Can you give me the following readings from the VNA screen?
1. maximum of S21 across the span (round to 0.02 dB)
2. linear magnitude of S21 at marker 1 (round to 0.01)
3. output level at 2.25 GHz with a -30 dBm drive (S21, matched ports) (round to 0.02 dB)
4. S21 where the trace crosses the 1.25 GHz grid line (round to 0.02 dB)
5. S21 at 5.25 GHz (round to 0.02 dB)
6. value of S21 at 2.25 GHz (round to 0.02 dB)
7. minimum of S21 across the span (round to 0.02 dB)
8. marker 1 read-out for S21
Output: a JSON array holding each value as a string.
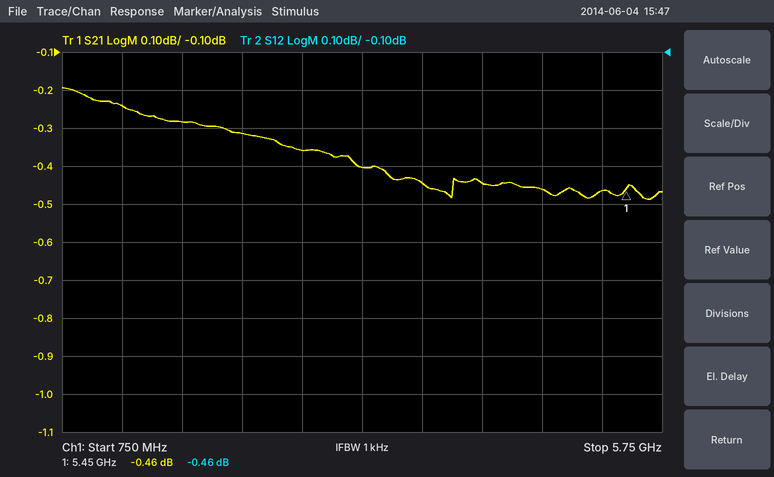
["-0.20 dB", "0.95", "-30.32 dBm", "-0.24 dB", "-0.46 dB", "-0.32 dB", "-0.48 dB", "-0.46 dB"]
